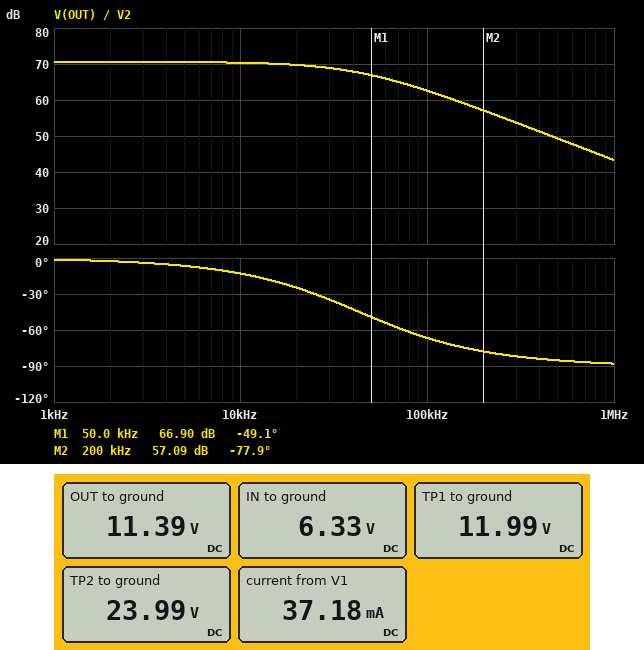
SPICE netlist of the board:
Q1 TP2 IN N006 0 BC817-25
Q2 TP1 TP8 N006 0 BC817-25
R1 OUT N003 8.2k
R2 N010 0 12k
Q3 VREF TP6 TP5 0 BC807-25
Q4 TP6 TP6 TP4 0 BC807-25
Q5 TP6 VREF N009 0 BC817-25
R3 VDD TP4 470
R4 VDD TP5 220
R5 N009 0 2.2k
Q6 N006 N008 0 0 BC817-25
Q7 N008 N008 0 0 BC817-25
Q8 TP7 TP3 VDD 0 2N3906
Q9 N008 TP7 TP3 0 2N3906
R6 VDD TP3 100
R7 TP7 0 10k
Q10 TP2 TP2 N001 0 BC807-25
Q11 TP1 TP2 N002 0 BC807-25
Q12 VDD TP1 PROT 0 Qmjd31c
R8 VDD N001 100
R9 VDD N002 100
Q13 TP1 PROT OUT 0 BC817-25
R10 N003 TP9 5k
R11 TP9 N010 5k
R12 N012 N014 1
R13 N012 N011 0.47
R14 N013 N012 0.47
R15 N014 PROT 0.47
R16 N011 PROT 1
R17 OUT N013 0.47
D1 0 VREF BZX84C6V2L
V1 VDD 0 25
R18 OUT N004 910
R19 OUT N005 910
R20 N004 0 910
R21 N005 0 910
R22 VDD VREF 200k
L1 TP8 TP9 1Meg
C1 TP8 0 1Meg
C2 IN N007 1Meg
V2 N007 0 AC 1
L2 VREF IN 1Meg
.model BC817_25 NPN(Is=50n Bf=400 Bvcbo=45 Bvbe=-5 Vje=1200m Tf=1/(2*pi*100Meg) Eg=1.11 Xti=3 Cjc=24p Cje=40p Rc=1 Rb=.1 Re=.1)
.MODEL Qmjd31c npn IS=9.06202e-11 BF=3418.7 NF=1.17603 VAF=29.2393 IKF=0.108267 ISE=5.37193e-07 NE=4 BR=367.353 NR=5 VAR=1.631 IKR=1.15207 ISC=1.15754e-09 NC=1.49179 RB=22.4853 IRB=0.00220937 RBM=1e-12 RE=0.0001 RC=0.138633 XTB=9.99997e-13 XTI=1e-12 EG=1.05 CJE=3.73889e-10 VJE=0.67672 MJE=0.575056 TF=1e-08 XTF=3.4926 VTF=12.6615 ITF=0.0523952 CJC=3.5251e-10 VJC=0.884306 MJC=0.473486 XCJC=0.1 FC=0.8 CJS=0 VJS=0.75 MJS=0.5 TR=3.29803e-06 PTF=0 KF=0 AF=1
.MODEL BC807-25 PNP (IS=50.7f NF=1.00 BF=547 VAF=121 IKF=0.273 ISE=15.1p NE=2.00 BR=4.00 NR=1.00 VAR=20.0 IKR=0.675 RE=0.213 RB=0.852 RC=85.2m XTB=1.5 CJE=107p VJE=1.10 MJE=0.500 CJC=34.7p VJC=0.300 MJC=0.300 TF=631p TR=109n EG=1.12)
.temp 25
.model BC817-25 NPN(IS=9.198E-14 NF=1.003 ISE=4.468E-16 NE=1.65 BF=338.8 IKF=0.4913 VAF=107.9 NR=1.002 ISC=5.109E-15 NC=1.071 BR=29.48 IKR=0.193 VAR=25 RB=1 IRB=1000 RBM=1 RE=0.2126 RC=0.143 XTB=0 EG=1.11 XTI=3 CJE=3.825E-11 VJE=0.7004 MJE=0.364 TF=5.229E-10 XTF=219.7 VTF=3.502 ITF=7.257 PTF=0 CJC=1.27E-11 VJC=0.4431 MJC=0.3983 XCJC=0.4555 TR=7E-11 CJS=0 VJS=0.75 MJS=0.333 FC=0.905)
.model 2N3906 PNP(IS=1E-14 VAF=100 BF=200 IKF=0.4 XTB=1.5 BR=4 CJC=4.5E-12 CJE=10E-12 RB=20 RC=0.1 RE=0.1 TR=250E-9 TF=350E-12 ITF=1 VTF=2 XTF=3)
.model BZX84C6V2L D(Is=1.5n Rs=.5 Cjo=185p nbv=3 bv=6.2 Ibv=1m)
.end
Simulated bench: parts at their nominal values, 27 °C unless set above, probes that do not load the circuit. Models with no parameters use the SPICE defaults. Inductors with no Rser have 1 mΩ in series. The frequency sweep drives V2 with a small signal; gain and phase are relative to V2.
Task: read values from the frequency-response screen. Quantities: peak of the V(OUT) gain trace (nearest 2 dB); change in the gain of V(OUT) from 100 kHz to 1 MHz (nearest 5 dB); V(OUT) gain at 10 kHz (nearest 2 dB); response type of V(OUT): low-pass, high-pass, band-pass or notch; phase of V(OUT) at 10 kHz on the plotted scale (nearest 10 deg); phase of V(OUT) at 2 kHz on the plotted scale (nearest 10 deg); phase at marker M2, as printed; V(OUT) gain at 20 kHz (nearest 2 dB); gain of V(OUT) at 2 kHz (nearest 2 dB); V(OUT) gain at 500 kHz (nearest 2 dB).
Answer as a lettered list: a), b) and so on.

a) 70 dB
b) -20 dB
c) 70 dB
d) low-pass
e) -10 deg
f) 0 deg
g) -77.9 deg
h) 70 dB
i) 70 dB
j) 50 dB
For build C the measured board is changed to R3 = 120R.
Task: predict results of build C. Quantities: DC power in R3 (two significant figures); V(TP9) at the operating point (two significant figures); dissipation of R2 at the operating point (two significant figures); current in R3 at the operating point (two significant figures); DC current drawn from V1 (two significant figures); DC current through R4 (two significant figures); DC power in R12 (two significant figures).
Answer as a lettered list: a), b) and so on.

a) 770 µW
b) 6.2 V
c) 1.6 mW
d) 2.5 mA
e) 33 mA
f) 1.5 mA
g) 40 µW
